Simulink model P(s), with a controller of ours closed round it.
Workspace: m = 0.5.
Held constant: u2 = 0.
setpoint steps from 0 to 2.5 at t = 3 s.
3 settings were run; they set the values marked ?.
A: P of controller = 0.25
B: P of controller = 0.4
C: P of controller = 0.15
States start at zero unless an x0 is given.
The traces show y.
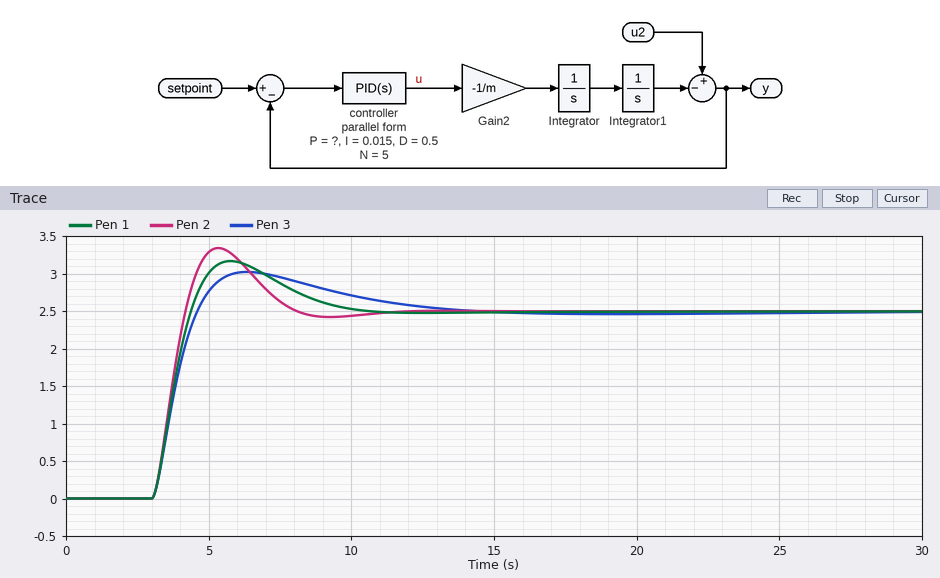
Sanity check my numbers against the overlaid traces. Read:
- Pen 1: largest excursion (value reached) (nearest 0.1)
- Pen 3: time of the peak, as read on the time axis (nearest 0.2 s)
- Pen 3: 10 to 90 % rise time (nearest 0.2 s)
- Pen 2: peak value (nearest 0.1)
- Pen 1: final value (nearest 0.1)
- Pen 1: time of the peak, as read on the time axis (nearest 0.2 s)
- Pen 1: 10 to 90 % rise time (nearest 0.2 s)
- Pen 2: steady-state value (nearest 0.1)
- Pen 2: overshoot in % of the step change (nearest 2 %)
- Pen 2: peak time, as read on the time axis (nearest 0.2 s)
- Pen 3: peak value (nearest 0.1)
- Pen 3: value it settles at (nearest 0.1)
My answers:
3.2
6.4 s
1.2 s
3.3
2.5
5.8 s
1.0 s
2.5
34 %
5.4 s
3.0
2.5
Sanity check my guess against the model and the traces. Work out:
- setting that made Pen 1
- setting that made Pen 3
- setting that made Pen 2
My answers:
A
C
B
